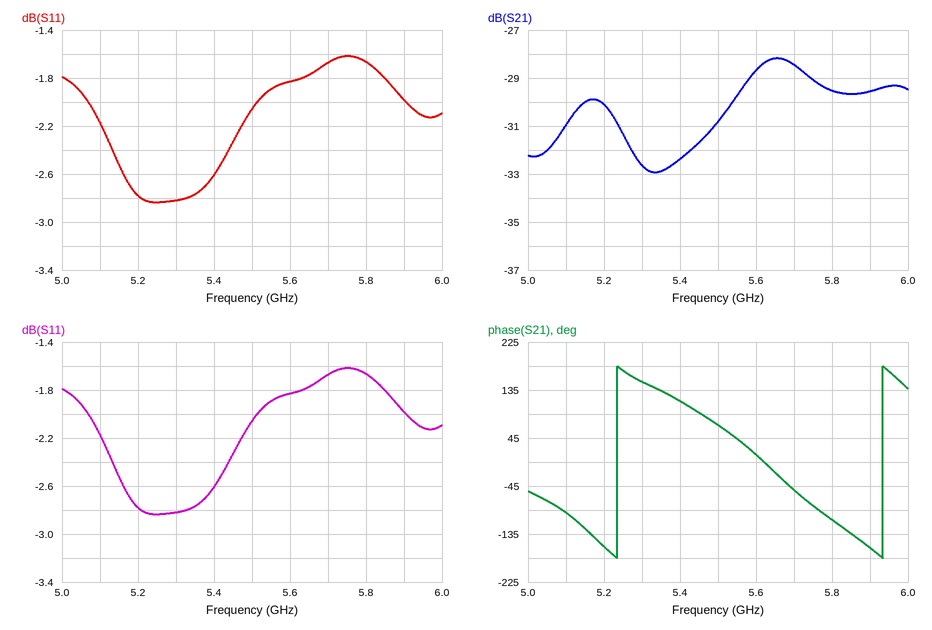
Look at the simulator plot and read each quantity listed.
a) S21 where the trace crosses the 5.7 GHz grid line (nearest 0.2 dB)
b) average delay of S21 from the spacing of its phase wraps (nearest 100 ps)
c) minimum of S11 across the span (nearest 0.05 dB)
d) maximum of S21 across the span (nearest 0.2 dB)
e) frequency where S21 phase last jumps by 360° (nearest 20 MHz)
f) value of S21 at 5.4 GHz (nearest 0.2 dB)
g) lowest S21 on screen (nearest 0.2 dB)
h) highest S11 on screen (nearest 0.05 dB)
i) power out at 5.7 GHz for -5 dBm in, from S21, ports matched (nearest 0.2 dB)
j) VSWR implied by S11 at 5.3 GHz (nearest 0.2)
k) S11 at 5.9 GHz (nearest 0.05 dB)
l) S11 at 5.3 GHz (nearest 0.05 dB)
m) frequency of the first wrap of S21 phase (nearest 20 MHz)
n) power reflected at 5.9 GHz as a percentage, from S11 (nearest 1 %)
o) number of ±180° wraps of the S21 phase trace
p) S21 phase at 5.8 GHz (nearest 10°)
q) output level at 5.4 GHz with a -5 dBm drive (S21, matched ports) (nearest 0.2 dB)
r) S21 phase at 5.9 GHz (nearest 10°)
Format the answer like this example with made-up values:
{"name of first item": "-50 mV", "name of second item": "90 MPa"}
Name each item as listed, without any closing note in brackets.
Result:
{"S21 where the trace crosses the 5.7 GHz grid line": "-28.4 dB", "average delay of S21 from the spacing of its phase wraps": "1.4 ns", "minimum of S11 across the span": "-2.85 dB", "maximum of S21 across the span": "-28.2 dB", "frequency where S21 phase last jumps by 360°": "5.94 GHz", "value of S21 at 5.4 GHz": "-32.4 dB", "lowest S21 on screen": "-33.0 dB", "highest S11 on screen": "-1.60 dB", "power out at 5.7 GHz for -5 dBm in, from S21, ports matched": "-33.4 dBm", "VSWR implied by S11 at 5.3 GHz": "6.2", "S11 at 5.9 GHz": "-2.00 dB", "S11 at 5.3 GHz": "-2.80 dB", "frequency of the first wrap of S21 phase": "5.24 GHz", "power reflected at 5.9 GHz as a percentage, from S11": "63 %", "number of ±180° wraps of the S21 phase trace": "2", "S21 phase at 5.8 GHz": "-110°", "output level at 5.4 GHz with a -5 dBm drive (S21, matched ports)": "-37.4 dBm", "S21 phase at 5.9 GHz": "-160°"}
